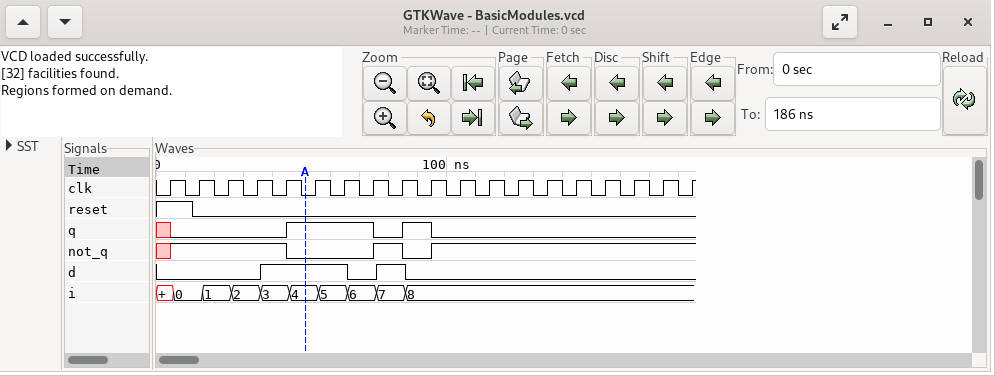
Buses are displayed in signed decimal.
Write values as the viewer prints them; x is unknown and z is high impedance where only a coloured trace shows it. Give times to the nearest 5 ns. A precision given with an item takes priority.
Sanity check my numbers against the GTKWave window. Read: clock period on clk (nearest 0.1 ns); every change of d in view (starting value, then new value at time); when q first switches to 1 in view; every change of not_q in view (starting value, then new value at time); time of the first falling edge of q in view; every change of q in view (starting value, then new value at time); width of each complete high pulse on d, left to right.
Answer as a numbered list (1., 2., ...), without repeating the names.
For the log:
1. 10 ns
2. 0, 1 at 35 ns, 0 at 65 ns, 1 at 75 ns, 0 at 85 ns
3. 45 ns
4. x, 1 at 5 ns, 0 at 45 ns, 1 at 75 ns, 0 at 85 ns, 1 at 95 ns
5. 75 ns
6. x, 0 at 5 ns, 1 at 45 ns, 0 at 75 ns, 1 at 85 ns, 0 at 95 ns
7. 30 ns, 10 ns
